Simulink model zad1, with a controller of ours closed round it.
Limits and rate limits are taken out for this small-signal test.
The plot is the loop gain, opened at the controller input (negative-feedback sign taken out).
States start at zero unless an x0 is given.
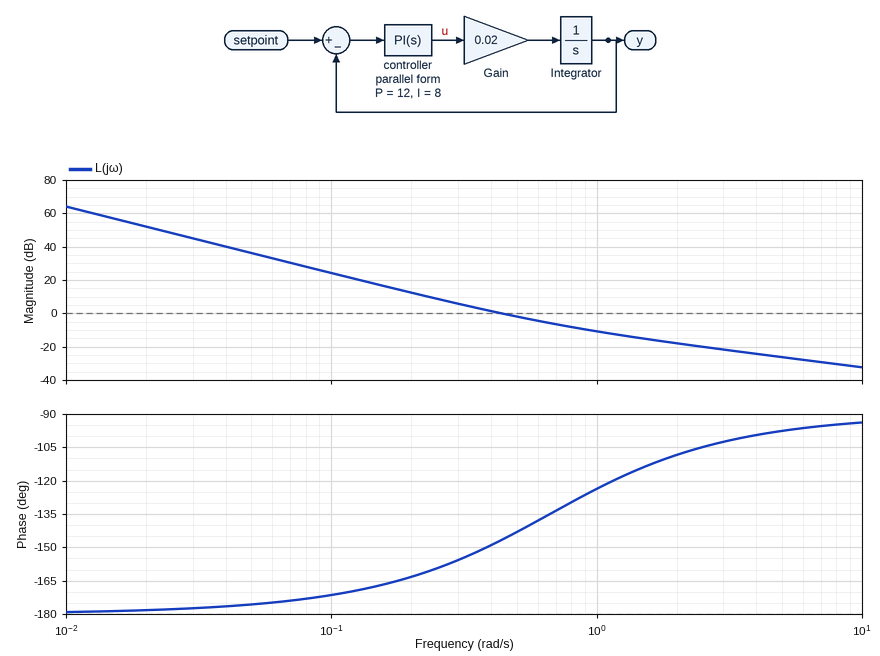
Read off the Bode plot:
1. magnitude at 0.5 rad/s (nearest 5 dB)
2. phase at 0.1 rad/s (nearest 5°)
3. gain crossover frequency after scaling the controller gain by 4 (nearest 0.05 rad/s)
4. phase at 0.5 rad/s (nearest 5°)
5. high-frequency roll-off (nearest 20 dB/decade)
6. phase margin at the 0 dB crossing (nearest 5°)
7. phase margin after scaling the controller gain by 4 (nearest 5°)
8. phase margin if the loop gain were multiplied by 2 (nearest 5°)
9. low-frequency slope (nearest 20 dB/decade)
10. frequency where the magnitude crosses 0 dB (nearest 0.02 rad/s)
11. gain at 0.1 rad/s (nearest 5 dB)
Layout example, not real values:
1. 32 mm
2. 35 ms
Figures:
1. 0 dB
2. -170°
3. 1.10 rad/s
4. -145°
5. -20 dB/decade
6. 35°
7. 60°
8. 45°
9. -40 dB/decade
10. 0.44 rad/s
11. 25 dB
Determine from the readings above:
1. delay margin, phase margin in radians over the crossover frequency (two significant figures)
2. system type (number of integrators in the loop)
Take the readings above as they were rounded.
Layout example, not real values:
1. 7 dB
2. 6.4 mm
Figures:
1. 1.4 s
2. 2
